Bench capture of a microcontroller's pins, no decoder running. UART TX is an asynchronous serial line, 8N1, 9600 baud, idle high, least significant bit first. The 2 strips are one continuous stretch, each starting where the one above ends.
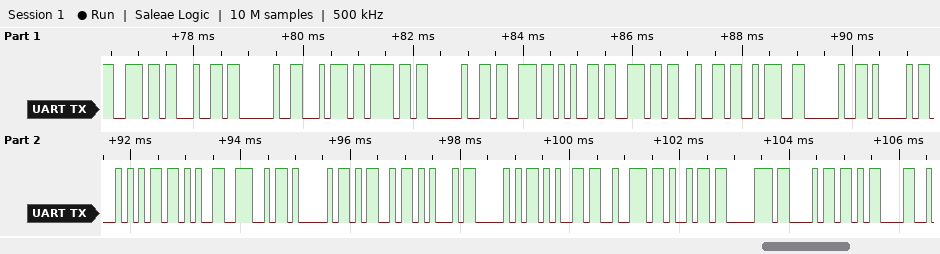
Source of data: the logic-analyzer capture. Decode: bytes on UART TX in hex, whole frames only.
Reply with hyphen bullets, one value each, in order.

- 6E 64 20 74 6F 20 73 65 6E 64 3A 20 41 54 2B 4E 41 4D 45 50 65 72 69 70 68 0D
